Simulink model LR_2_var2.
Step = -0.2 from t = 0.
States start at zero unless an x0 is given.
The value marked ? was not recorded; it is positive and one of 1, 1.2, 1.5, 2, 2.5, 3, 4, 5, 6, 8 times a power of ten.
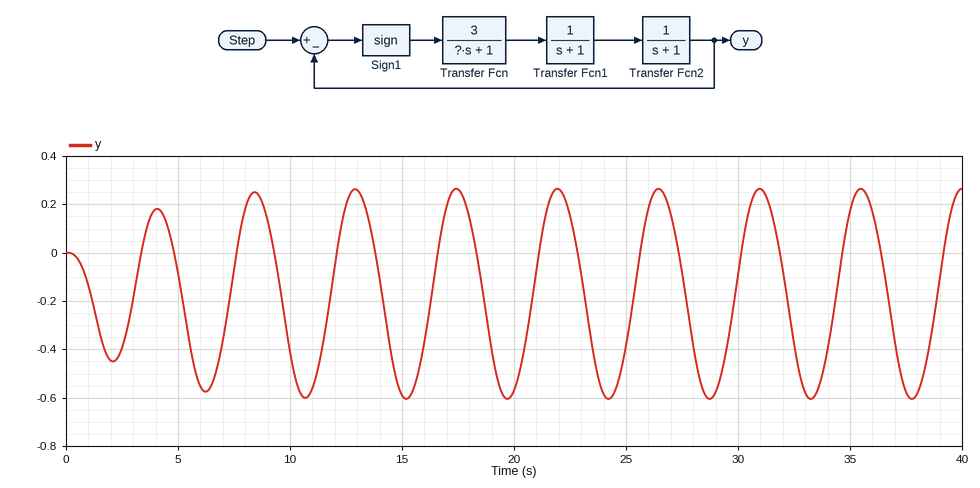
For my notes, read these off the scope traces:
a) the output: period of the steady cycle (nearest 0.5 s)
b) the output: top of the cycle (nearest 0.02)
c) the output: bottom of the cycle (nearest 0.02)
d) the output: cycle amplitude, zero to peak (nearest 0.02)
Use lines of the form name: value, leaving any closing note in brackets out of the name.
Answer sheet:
the output: period of the steady cycle: 4.5 s
the output: top of the cycle: 0.26
the output: bottom of the cycle: -0.60
the output: cycle amplitude, zero to peak: 0.44
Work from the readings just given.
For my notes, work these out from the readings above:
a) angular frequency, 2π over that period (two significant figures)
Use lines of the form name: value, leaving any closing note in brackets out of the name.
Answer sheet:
angular frequency, 2π over that period: 1.4 rad/s
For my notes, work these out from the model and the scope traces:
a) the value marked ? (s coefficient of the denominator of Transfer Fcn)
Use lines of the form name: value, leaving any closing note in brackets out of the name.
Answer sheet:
the value marked ?: 2
